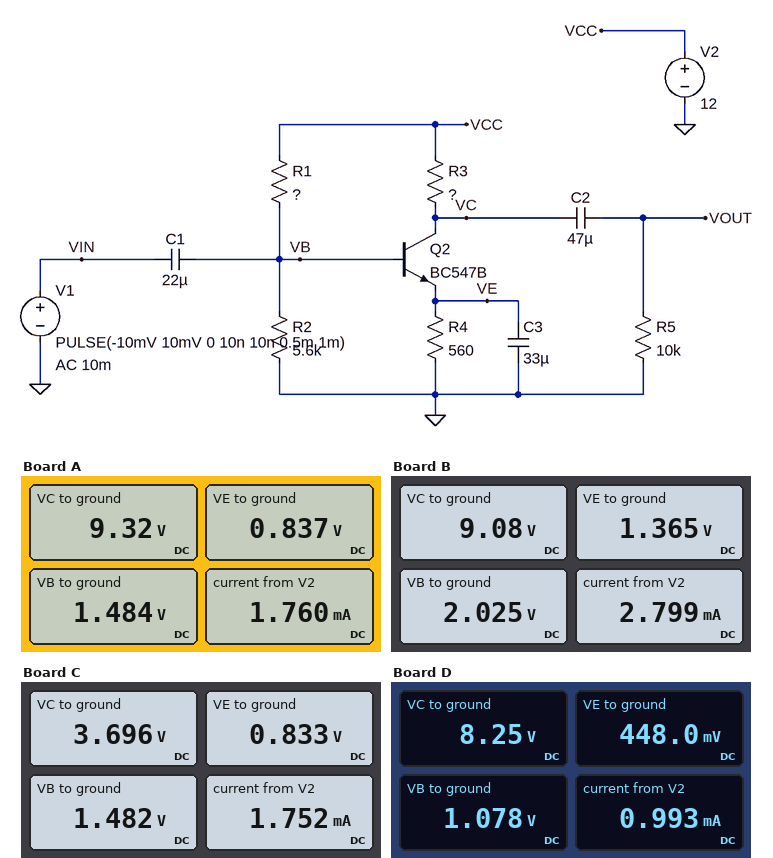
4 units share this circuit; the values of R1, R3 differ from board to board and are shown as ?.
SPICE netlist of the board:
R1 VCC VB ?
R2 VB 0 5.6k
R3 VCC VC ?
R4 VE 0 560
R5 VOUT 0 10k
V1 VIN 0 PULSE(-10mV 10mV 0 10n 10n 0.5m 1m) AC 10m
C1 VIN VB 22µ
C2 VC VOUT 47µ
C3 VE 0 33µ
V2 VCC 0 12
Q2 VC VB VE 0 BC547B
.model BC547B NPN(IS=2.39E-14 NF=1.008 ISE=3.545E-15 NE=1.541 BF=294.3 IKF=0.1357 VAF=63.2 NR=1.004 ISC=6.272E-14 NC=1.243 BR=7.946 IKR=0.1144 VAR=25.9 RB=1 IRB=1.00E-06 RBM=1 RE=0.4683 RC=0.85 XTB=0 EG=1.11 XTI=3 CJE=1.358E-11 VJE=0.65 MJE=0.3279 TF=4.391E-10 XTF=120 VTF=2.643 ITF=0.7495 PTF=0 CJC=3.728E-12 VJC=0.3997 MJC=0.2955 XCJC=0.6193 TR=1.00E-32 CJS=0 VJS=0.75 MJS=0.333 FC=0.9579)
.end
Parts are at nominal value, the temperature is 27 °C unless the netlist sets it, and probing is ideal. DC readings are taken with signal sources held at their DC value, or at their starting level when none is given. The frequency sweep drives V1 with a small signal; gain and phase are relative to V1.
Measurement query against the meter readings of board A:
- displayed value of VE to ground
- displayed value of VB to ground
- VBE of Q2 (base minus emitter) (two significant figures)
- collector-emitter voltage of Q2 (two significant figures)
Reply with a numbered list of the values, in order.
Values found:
1. 0.837 V
2. 1.484 V
3. 650 mV
4. 8.5 V
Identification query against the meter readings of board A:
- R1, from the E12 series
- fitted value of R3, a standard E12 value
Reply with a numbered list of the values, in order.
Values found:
1. 39 kΩ
2. 1.8 kΩ
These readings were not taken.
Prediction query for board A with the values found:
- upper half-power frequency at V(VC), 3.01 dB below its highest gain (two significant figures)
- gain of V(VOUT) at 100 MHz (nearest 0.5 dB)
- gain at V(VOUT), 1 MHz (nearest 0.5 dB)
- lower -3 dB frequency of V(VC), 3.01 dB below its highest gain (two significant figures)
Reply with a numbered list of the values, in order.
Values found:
1. 68 MHz
2. 33.0 dB
3. 38.0 dB
4. 270 Hz
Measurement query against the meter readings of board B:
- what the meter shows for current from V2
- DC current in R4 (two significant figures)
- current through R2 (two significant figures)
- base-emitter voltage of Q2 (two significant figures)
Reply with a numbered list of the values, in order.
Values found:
1. 2.799 mA
2. 2.4 mA
3. 360 µA
4. 660 mV
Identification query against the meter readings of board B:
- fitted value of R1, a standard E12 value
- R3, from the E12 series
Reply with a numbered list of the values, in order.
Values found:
1. 27 kΩ
2. 1.2 kΩ
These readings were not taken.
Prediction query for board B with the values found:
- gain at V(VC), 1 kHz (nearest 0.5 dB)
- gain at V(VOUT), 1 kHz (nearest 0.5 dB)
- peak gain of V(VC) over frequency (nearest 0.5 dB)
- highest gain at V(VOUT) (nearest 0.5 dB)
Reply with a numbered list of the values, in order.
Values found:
1. 38.5 dB
2. 38.5 dB
3. 39.0 dB
4. 39.0 dB
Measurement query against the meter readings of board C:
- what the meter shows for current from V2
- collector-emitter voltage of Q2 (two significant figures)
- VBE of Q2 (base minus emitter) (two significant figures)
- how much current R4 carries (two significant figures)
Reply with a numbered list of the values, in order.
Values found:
1. 1.752 mA
2. 2.9 V
3. 650 mV
4. 1.5 mA
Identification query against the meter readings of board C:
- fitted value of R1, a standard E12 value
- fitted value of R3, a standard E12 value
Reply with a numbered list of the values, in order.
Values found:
1. 39 kΩ
2. 5.6 kΩ
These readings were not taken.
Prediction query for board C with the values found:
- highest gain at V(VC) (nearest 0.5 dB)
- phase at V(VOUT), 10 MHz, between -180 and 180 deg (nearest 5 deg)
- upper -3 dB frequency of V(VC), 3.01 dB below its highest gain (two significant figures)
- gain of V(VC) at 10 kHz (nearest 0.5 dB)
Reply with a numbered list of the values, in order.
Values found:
1. 45.0 dB
2. 155 deg
3. 22 MHz
4. 45.0 dB
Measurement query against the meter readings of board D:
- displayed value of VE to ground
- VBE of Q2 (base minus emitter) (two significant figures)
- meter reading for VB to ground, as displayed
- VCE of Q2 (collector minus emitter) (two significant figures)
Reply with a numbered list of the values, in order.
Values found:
1. 448.0 mV
2. 630 mV
3. 1.078 V
4. 7.8 V
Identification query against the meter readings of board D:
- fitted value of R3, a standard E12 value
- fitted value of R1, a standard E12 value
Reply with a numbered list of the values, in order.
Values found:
1. 4.7 kΩ
2. 56 kΩ
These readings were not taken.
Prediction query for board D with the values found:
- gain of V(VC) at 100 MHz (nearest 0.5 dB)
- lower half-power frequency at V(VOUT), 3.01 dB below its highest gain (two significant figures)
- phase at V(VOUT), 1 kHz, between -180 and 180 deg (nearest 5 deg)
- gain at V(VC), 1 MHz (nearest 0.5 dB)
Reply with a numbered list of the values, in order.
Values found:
1. 29.0 dB
2. 150 Hz
3. -170 deg
4. 39.5 dB
